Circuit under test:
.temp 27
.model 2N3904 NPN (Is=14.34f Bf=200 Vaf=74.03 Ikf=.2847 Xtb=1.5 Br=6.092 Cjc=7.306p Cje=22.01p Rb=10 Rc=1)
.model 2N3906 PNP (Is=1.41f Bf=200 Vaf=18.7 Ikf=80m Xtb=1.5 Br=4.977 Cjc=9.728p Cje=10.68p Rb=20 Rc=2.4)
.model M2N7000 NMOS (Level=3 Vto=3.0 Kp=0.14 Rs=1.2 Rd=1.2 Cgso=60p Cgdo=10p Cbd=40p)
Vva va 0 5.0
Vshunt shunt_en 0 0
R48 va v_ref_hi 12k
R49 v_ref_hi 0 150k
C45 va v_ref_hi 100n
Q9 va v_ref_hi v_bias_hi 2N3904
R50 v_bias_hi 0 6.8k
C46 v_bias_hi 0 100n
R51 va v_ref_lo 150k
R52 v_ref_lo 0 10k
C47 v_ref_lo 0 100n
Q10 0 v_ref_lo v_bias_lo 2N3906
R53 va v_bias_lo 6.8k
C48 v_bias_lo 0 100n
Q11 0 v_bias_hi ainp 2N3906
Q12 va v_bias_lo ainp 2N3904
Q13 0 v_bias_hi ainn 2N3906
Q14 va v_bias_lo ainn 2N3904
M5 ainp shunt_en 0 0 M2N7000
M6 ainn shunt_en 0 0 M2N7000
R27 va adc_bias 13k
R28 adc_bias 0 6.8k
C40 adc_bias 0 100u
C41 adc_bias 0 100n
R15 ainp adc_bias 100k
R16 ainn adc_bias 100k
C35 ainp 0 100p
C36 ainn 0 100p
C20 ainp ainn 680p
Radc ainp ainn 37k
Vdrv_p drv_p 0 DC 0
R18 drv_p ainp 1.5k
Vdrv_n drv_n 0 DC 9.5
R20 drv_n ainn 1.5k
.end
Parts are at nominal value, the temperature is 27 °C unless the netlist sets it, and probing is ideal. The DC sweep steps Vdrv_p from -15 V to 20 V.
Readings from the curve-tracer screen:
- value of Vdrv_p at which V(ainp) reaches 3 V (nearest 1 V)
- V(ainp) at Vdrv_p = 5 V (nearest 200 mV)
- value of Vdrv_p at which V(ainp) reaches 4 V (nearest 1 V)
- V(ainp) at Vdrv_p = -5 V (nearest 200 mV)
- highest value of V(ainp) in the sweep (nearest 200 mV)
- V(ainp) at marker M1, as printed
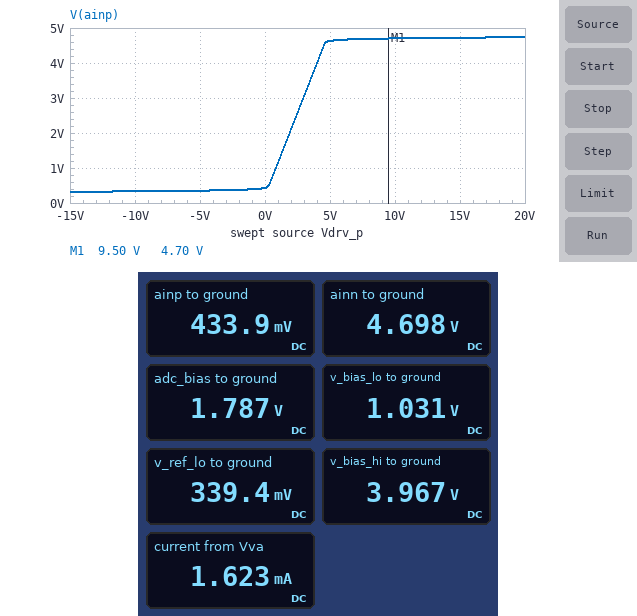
3 V
4.6 V
4 V
400 mV
4.8 V
4.70 V
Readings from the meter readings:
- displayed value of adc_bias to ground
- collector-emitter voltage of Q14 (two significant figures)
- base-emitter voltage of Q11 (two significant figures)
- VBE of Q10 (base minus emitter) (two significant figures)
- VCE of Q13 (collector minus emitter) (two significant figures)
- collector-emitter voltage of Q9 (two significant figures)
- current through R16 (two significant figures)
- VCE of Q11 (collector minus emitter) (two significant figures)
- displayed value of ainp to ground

1.787 V
300 mV
3.5 V
-690 mV
-4.7 V
1.0 V
29 µA
-430 mV
433.9 mV
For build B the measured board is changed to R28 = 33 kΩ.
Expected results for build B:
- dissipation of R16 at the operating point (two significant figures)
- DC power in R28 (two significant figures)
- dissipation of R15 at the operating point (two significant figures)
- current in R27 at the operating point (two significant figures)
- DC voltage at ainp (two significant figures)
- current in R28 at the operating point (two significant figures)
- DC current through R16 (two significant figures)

16 µW
360 µW
89 µW
120 µA
440 mV
100 µA
13 µA
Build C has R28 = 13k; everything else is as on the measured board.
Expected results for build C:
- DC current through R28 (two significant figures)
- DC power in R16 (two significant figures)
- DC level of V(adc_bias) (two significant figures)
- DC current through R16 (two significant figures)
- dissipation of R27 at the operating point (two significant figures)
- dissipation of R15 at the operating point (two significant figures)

190 µA
48 µW
2.5 V
22 µA
480 µW
43 µW
